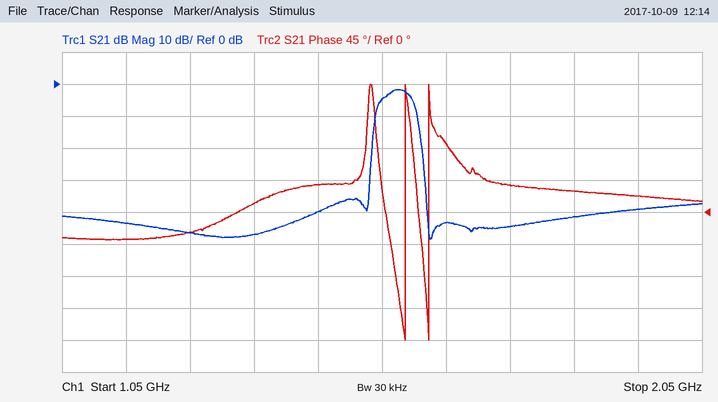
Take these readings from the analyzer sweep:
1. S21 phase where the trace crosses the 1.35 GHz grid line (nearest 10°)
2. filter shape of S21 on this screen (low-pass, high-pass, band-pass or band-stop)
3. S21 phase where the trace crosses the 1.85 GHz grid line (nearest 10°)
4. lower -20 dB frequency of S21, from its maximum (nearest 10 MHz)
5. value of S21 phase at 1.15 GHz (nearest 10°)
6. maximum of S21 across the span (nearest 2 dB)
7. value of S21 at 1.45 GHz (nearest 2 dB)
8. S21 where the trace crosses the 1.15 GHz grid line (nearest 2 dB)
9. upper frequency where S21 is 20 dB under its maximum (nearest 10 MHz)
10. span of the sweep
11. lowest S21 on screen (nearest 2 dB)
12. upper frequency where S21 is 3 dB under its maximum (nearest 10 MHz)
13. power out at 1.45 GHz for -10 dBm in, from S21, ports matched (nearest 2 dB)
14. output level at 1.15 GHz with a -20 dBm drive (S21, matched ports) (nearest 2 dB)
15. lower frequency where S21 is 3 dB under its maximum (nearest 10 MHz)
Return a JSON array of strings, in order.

["10°", "band-pass", "30°", "1.53 GHz", "-40°", "-2 dB", "-40 dB", "-44 dB", "1.61 GHz", "1 GHz", "-48 dB", "1.60 GHz", "-50 dBm", "-64 dBm", "1.55 GHz"]
